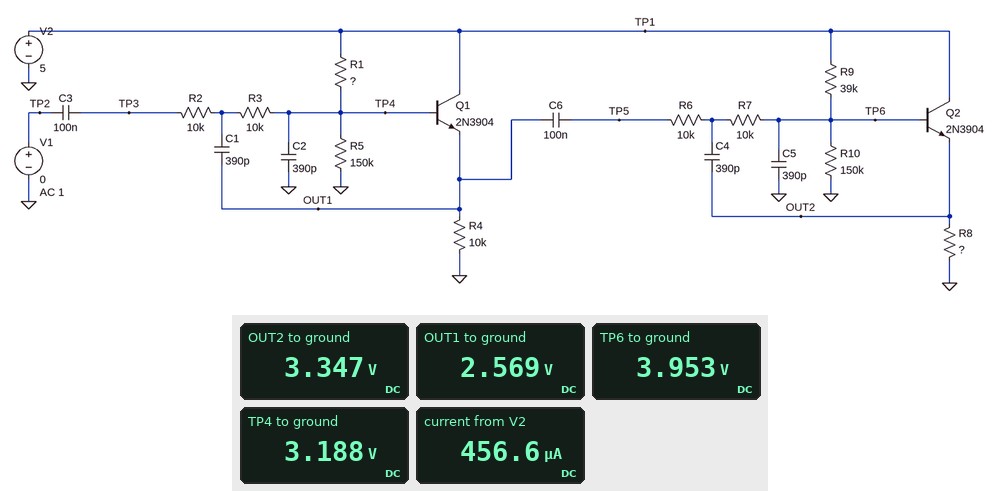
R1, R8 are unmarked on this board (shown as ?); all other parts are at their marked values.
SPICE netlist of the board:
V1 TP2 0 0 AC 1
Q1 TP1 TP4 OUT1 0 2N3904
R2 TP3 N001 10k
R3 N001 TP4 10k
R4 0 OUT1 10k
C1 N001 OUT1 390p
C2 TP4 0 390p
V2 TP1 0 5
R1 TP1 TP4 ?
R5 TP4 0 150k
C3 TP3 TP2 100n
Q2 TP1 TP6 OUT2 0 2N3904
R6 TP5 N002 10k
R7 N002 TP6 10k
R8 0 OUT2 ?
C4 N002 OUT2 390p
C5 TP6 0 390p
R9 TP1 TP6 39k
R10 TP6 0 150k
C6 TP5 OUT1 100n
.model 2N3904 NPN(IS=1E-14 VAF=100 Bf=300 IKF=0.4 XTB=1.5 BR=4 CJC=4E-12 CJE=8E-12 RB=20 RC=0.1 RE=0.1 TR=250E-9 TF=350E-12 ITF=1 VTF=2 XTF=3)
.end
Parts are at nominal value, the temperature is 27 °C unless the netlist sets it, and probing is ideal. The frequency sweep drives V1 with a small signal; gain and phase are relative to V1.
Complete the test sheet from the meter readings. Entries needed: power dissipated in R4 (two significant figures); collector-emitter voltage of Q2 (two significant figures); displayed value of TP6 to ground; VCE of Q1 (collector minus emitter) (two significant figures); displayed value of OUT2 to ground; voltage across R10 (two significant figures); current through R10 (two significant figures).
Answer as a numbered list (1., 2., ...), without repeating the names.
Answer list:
1. 660 µW
2. 1.7 V
3. 3.953 V
4. 2.4 V
5. 3.347 V
6. 4.0 V
7. 26 µA
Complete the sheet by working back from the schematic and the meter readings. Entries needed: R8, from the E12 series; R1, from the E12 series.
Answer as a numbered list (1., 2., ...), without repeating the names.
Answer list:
1. 22 kΩ
2. 82 kΩ
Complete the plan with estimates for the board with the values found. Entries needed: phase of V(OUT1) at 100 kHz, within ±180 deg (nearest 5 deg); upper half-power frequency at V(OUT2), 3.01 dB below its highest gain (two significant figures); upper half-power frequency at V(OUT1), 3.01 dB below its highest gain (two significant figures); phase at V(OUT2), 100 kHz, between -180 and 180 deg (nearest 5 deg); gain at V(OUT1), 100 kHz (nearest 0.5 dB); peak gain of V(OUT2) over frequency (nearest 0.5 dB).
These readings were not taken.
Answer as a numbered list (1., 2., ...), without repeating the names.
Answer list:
1. -130 deg
2. 24 kHz
3. 33 kHz
4. 105 deg
5. -18.0 dB
6. -7.5 dB
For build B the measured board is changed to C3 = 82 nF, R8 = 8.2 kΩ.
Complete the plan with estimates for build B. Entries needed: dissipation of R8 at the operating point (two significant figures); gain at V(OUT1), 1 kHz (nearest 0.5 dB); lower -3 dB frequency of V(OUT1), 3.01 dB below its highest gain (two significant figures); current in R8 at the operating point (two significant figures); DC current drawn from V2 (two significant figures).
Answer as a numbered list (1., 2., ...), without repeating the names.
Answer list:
1. 1.3 mW
2. -3.0 dB
3. 27 Hz
4. 400 µA
5. 710 µA
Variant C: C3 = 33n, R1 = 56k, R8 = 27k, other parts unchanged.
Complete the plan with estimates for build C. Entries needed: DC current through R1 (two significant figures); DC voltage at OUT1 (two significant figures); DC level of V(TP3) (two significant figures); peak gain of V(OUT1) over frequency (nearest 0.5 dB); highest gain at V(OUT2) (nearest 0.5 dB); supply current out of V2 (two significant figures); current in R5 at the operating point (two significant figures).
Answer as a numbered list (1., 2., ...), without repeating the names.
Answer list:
1. 25 µA
2. 3.0 V
3. 3.6 V
4. -3.5 dB
5. -8.0 dB
6. 470 µA
7. 24 µA
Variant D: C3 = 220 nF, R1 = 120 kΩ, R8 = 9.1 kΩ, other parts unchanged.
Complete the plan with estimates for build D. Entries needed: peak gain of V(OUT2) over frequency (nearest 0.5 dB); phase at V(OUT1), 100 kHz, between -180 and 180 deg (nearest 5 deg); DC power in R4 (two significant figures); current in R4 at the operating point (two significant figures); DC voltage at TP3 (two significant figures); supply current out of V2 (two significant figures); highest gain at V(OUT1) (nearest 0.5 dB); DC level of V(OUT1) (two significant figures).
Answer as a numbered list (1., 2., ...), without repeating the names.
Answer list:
1. -7.0 dB
2. -130 deg
3. 450 µW
4. 210 µA
5. 2.7 V
6. 620 µA
7. -2.5 dB
8. 2.1 V
